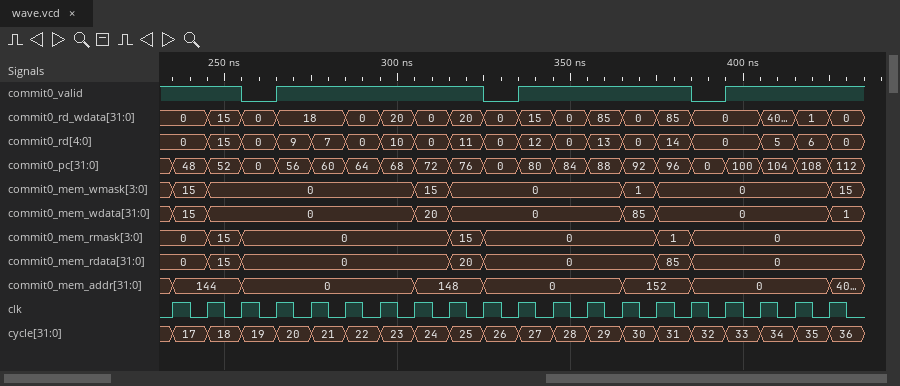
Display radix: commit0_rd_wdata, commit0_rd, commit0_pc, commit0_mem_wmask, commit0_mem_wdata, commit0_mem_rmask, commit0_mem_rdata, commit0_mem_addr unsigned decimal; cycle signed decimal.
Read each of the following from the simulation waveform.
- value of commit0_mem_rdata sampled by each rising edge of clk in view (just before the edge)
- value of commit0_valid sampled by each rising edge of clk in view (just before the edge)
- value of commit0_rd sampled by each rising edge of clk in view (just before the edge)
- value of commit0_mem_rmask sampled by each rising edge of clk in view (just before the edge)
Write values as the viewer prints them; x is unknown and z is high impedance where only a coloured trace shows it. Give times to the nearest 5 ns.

0, 0, 15, 0, 0, 0, 0, 0, 0, 20, 0, 0, 0, 0, 0, 85, 0, 0, 0, 0
1 1 1 0 1 1 1 1 1 1 0 1 1 1 1 1 0 1 1 1
0, 0, 15, 0, 9, 7, 0, 10, 0, 11, 0, 12, 0, 13, 0, 14, 0, 0, 5, 6
0, 0, 15, 0, 0, 0, 0, 0, 0, 15, 0, 0, 0, 0, 0, 1, 0, 0, 0, 0
